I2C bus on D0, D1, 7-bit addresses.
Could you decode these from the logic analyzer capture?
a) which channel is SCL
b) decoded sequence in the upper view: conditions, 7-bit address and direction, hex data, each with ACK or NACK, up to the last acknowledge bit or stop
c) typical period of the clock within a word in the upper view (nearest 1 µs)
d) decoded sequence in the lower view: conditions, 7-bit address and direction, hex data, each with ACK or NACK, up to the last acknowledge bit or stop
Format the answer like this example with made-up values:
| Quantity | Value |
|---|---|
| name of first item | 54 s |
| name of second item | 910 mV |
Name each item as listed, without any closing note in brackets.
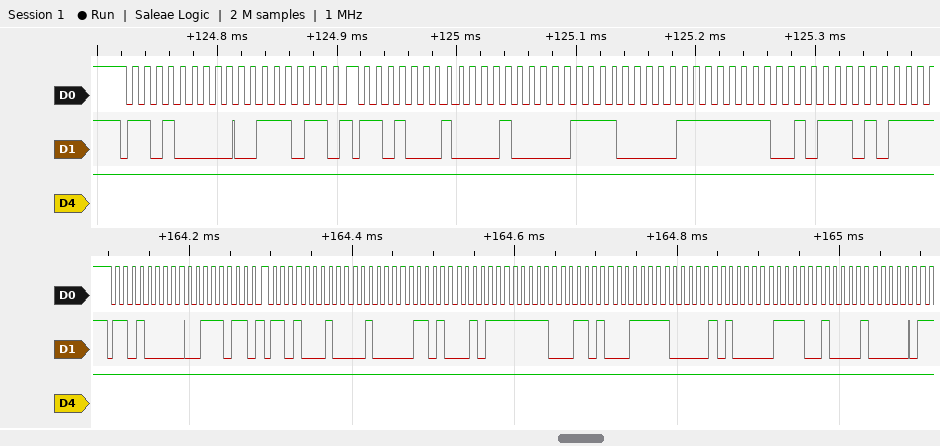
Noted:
| Quantity | Value |
|---|---|
| which channel is SCL | D0 |
| decoded sequence in the upper view: conditions, 7-bit address and direction, hex data, each with ACK or NACK, up to the last acknowledge bit or stop | start, address 68 write ACK, 3B ACK, repeated start, address 68 read ACK, 10 ACK, F0 ACK, FF ACK, 5D ACK |
| typical period of the clock within a word in the upper view | 10 µs |
| decoded sequence in the lower view: conditions, 7-bit address and direction, hex data, each with ACK or NACK, up to the last acknowledge bit or stop | start, address 68 write ACK, 3B ACK, repeated start, address 68 read ACK, 10 ACK, D1 ACK, FF ACK, 34 ACK, F8 ACK, 50 ACK, F2 ACK, 20 ACK |
